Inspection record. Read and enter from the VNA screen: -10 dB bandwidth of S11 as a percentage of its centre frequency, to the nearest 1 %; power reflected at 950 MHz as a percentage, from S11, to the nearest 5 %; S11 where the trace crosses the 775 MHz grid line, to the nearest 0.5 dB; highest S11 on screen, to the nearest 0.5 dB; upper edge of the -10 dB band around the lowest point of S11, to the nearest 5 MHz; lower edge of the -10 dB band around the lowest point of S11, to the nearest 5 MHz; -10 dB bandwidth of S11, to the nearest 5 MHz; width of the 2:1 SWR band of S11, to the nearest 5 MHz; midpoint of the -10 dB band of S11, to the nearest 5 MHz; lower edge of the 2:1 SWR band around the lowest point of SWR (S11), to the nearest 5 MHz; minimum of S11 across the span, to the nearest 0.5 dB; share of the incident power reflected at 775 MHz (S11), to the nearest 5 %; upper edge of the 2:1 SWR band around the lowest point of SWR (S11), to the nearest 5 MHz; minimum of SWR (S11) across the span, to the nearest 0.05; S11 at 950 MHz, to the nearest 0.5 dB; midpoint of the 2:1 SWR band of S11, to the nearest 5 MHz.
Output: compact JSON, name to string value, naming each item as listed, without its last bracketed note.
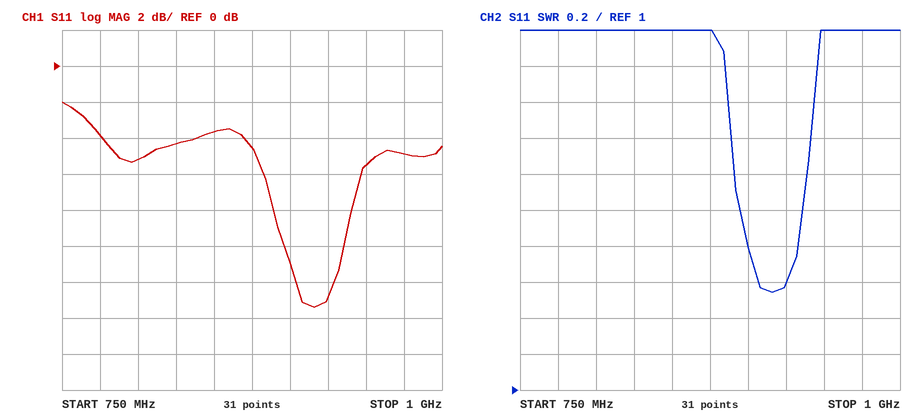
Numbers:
{"-10 dB bandwidth of S11 as a percentage of its centre frequency, to the nearest 1 %": "4 %", "power reflected at 950 MHz as a percentage, from S11, to the nearest 5 %": "30 %", "S11 where the trace crosses the 775 MHz grid line, to the nearest 0.5 dB": "-4.0 dB", "highest S11 on screen, to the nearest 0.5 dB": "-2.0 dB", "upper edge of the -10 dB band around the lowest point of S11, to the nearest 5 MHz": "935 MHz", "lower edge of the -10 dB band around the lowest point of S11, to the nearest 5 MHz": "895 MHz", "-10 dB bandwidth of S11, to the nearest 5 MHz": "40 MHz", "width of the 2:1 SWR band of S11, to the nearest 5 MHz": "40 MHz", "midpoint of the -10 dB band of S11, to the nearest 5 MHz": "915 MHz", "lower edge of the 2:1 SWR band around the lowest point of SWR (S11), to the nearest 5 MHz": "895 MHz", "minimum of S11 across the span, to the nearest 0.5 dB": "-13.5 dB", "share of the incident power reflected at 775 MHz (S11), to the nearest 5 %": "40 %", "upper edge of the 2:1 SWR band around the lowest point of SWR (S11), to the nearest 5 MHz": "935 MHz", "minimum of SWR (S11) across the span, to the nearest 0.05": "1.55", "S11 at 950 MHz, to the nearest 0.5 dB": "-5.5 dB", "midpoint of the 2:1 SWR band of S11, to the nearest 5 MHz": "915 MHz"}
